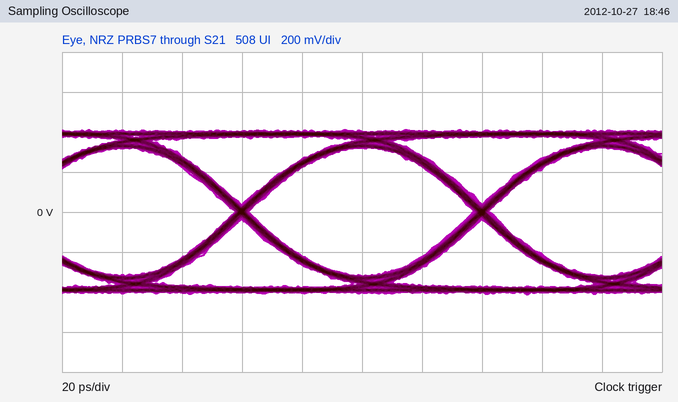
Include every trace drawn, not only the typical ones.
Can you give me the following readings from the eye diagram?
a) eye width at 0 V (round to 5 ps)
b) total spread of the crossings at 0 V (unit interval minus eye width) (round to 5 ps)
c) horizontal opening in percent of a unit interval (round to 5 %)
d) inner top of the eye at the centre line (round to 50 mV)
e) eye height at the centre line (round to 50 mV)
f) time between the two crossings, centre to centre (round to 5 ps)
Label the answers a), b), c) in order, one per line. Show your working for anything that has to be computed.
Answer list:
a) 75 ps
b) 5 ps
c) 75 ps / 80 ps ≈ 93.8 %, so 95 % to the nearest 5 %
d) 300 mV
e) 650 mV
f) 80 ps
